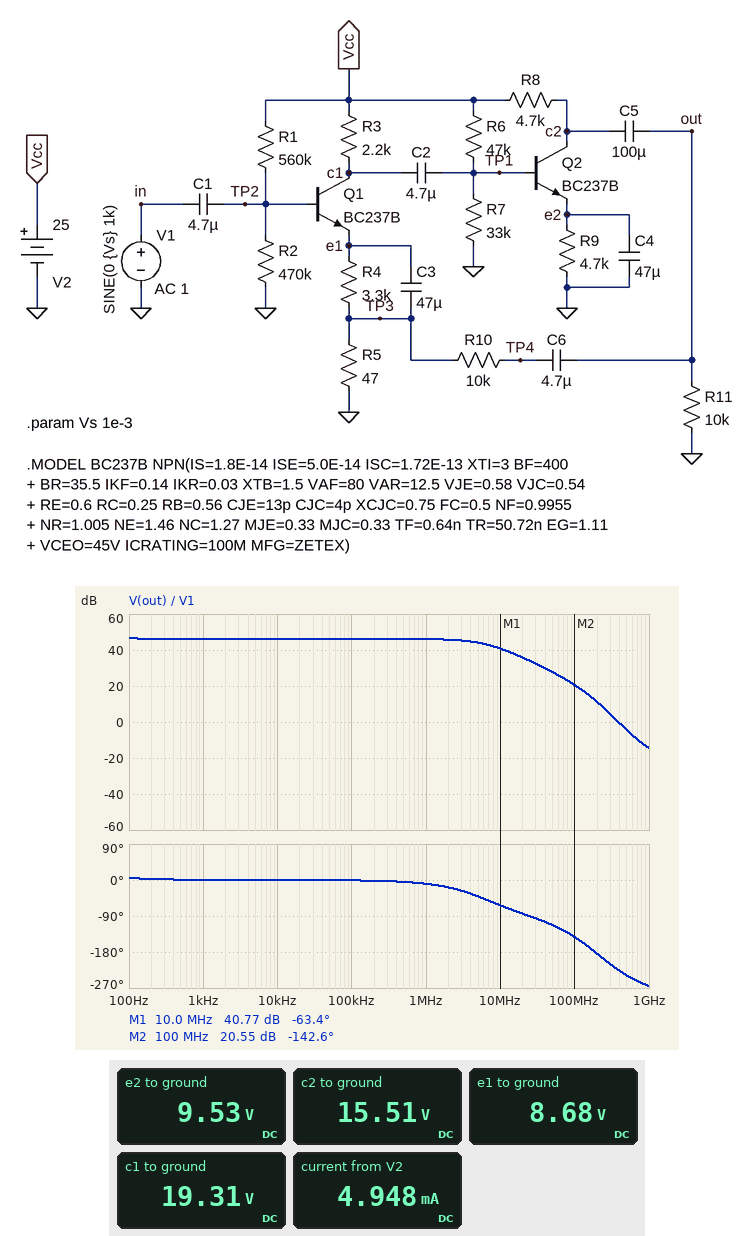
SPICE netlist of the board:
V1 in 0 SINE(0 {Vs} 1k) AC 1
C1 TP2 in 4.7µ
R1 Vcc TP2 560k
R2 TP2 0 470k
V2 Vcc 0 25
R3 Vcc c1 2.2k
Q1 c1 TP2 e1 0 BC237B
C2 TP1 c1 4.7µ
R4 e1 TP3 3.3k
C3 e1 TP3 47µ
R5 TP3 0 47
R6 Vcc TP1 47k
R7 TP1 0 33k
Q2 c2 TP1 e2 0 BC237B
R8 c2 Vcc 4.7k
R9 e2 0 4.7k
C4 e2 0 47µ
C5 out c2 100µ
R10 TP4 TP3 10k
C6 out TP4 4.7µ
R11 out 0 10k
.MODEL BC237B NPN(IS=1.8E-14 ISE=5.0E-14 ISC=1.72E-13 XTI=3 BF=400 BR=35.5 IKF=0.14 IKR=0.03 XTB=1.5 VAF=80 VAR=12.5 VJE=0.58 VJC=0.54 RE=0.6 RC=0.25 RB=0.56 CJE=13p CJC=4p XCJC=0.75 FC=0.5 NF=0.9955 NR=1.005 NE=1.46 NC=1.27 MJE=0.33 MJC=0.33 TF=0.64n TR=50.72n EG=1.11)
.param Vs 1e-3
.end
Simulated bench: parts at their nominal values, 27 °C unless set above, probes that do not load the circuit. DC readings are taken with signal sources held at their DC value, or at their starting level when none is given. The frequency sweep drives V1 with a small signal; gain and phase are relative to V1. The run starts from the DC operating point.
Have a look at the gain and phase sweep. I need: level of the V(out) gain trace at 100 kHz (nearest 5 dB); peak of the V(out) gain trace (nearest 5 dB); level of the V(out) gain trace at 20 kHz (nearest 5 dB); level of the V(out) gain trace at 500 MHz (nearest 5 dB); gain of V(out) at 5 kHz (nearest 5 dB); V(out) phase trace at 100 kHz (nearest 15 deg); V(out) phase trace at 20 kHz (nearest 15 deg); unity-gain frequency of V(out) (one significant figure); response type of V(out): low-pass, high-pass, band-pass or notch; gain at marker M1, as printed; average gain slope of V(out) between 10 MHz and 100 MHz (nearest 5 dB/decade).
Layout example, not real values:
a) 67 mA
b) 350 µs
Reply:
a) 45 dB
b) 45 dB
c) 45 dB
d) -5 dB
e) 45 dB
f) 0 deg
g) 0 deg
h) 400 MHz
i) low-pass
j) 40.77 dB
k) -20 dB/decade
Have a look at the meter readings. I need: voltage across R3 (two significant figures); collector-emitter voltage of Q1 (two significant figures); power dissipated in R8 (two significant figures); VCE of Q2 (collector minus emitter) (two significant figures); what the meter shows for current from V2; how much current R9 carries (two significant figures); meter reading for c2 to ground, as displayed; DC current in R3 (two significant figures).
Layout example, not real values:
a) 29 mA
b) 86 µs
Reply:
a) 5.7 V
b) 11 V
c) 19 mW
d) 6.0 V
e) 4.948 mA
f) 2.0 mA
g) 15.51 V
h) 2.6 mA
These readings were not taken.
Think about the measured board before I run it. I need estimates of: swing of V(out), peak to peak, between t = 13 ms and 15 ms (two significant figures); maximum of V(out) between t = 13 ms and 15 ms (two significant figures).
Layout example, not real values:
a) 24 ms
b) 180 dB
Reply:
a) 410 mV
b) 200 mV
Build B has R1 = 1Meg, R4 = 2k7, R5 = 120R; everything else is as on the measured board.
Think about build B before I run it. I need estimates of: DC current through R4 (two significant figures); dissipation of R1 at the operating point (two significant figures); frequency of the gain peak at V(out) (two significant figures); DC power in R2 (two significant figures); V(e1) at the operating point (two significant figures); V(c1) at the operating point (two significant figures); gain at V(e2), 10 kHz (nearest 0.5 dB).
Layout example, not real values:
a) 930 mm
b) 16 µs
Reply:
a) 1.9 mA
b) 360 µW
c) 16 Hz
d) 80 µW
e) 5.5 V
f) 21 V
g) -39.0 dB
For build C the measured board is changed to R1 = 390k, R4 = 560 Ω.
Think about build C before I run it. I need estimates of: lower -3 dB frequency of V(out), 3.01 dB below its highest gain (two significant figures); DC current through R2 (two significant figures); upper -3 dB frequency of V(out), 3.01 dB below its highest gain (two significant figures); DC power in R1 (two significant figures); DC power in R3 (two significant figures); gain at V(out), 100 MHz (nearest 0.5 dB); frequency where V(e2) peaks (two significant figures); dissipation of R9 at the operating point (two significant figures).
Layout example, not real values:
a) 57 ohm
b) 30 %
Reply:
a) 42 Hz
b) 13 µA
c) 79 Hz
d) 920 µW
e) 170 mW
f) 28.5 dB
g) 49 Hz
h) 19 mW
